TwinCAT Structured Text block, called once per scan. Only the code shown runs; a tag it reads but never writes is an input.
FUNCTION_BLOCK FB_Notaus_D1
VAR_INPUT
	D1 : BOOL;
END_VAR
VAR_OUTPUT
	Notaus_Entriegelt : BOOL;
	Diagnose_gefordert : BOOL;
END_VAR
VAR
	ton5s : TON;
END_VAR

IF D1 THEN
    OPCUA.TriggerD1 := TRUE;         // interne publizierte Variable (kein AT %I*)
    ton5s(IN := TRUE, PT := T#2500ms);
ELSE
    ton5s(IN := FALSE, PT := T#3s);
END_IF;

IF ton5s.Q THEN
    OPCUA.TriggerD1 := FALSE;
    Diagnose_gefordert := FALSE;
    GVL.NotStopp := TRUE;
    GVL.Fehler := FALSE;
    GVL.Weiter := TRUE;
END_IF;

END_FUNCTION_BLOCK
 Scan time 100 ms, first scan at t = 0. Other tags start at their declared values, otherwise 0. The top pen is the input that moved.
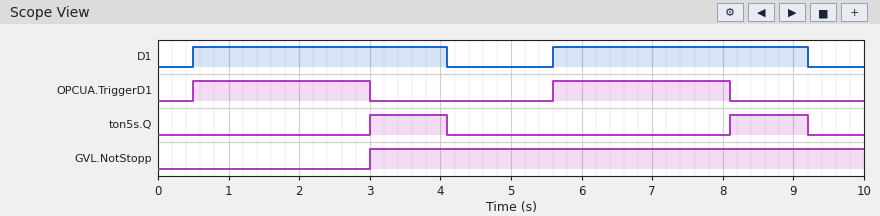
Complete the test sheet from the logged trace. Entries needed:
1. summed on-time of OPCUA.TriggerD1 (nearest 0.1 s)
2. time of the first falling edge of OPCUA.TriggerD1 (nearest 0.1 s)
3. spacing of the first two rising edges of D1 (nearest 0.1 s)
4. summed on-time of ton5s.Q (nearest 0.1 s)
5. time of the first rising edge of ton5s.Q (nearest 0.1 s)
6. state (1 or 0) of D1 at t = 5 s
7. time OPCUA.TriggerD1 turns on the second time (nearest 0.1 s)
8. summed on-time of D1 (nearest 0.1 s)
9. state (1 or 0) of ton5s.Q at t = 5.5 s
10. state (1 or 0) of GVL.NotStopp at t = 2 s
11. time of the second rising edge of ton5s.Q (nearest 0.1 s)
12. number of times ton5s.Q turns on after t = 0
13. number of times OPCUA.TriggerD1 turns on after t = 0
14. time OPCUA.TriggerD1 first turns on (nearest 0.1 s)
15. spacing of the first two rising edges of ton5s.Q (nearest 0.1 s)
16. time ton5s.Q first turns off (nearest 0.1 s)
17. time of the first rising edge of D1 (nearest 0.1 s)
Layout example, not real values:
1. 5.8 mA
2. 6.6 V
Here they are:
1. 5.0 s
2. 3.0 s
3. 5.1 s
4. 2.2 s
5. 3.0 s
6. 0
7. 5.6 s
8. 7.2 s
9. 0
10. 0
11. 8.1 s
12. 2
13. 2
14. 0.5 s
15. 5.1 s
16. 4.1 s
17. 0.5 s
